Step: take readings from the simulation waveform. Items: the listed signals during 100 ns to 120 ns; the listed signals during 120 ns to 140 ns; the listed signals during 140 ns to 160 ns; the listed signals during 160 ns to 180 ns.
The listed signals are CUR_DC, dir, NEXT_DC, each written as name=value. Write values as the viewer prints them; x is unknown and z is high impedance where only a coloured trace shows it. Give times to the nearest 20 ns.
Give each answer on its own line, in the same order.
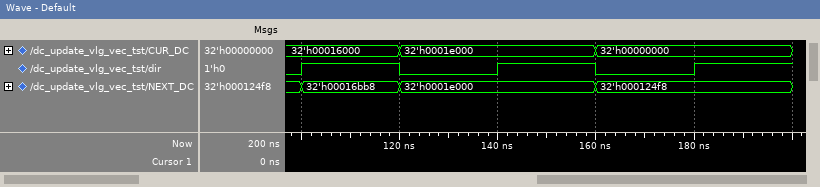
CUR_DC=32'h00016000, dir=1, NEXT_DC=32'h00016bb8
CUR_DC=32'h0001e000, dir=0, NEXT_DC=32'h0001e000
CUR_DC=32'h0001e000, dir=1, NEXT_DC=32'h0001e000
CUR_DC=32'h00000000, dir=0, NEXT_DC=32'h000124f8
